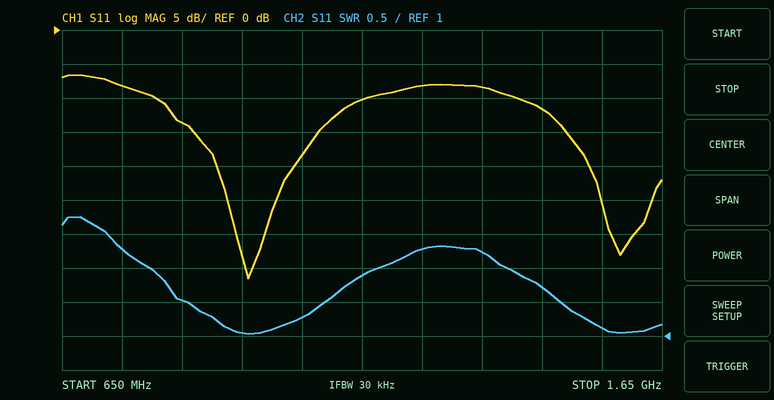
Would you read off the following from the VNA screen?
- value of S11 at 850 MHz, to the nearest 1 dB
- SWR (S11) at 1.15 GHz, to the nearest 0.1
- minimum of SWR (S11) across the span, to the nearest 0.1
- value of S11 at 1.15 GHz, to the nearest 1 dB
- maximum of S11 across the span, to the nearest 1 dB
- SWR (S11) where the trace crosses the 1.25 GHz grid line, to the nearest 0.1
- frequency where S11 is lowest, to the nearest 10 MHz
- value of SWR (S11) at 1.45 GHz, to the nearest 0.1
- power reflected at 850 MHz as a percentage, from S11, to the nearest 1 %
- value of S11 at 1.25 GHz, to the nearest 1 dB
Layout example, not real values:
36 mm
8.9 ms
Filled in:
-14 dB
1.9
1.0
-10 dB
-7 dB
2.3
960 MHz
1.7
4 %
-8 dB
